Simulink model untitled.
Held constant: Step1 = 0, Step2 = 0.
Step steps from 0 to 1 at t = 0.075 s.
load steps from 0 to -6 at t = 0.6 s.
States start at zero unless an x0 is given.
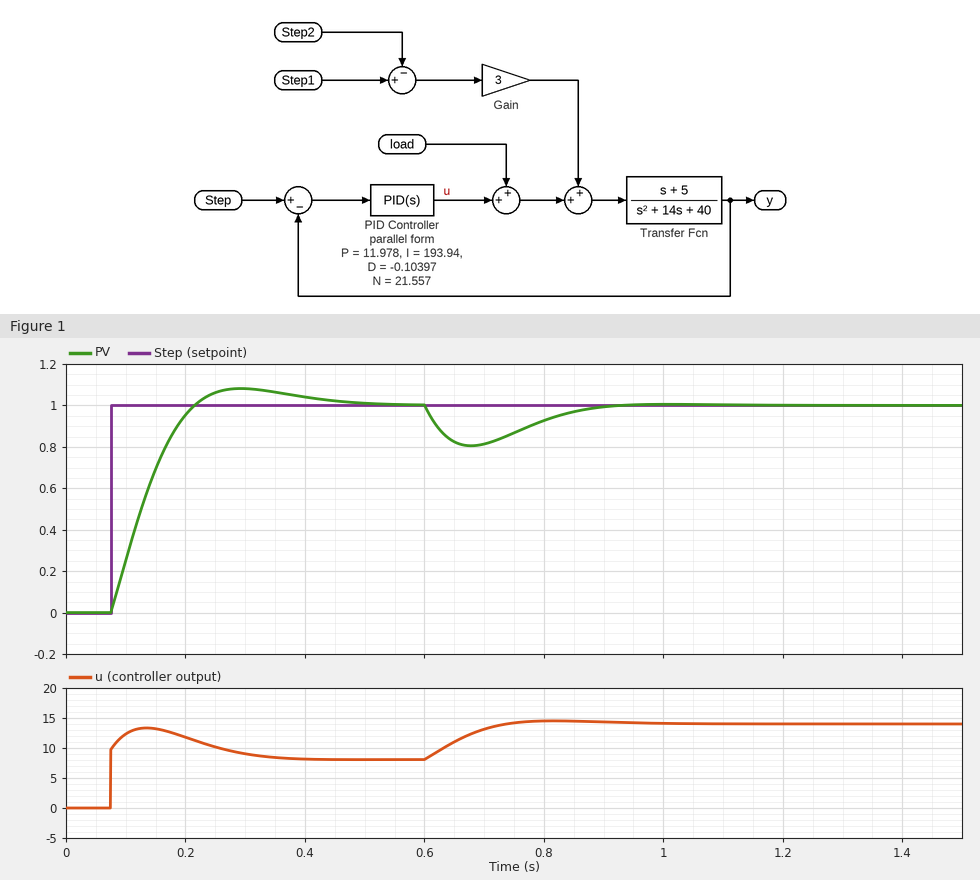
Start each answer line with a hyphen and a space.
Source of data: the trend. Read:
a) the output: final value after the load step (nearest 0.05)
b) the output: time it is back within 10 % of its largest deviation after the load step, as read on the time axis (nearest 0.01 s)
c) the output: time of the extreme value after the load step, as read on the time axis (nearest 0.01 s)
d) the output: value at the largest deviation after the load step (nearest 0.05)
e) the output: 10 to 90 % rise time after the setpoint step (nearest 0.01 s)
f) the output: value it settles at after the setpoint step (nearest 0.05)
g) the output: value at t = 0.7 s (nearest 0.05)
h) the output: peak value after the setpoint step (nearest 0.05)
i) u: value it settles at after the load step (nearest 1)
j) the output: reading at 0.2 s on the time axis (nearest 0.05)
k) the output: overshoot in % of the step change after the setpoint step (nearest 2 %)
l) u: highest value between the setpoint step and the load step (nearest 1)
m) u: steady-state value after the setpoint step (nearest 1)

- 1.00
- 0.87 s
- 0.68 s
- 0.80
- 0.10 s
- 1.00
- 0.80
- 1.10
- 14
- 0.95
- 8 %
- 13
- 8
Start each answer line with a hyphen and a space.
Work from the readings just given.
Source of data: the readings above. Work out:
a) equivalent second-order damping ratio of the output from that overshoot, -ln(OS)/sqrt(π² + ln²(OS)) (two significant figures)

- 0.63
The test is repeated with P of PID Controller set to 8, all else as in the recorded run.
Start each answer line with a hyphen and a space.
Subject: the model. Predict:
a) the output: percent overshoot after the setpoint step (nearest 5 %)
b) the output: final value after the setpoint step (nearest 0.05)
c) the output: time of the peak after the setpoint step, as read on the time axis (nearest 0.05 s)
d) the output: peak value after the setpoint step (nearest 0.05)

- 15 %
- 1.00
- 0.30 s
- 1.15
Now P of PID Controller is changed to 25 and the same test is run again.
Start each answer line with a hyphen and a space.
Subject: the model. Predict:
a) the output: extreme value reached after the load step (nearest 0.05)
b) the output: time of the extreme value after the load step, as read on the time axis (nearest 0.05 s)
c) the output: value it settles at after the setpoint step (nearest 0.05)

- 0.85
- 0.65 s
- 1.00
